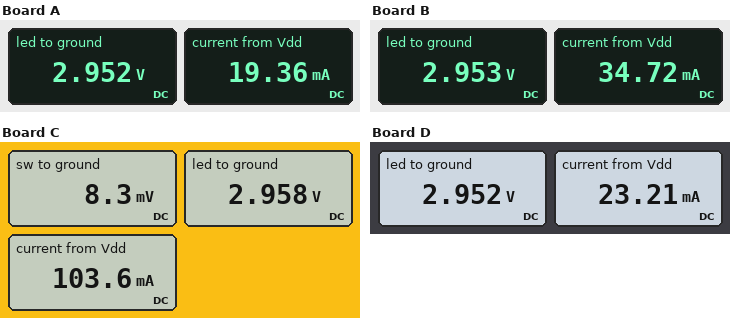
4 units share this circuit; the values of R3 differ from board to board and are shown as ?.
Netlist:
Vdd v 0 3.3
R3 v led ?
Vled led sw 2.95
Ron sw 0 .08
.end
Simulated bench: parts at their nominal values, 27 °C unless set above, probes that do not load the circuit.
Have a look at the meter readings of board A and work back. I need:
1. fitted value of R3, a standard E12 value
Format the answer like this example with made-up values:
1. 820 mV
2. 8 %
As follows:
1. 18 Ω
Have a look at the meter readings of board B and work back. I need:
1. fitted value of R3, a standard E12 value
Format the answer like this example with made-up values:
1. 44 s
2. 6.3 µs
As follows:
1. 10 Ω
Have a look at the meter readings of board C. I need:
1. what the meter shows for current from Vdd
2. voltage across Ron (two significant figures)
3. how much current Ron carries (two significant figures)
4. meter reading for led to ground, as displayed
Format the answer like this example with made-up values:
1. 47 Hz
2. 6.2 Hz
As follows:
1. 103.6 mA
2. 8.3 mV
3. 100 mA
4. 2.958 V
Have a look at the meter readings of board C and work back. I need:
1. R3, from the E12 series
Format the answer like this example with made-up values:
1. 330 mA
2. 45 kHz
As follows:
1. 3.3 Ω
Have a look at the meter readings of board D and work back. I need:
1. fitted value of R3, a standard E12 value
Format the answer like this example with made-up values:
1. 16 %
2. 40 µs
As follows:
1. 15 Ω
